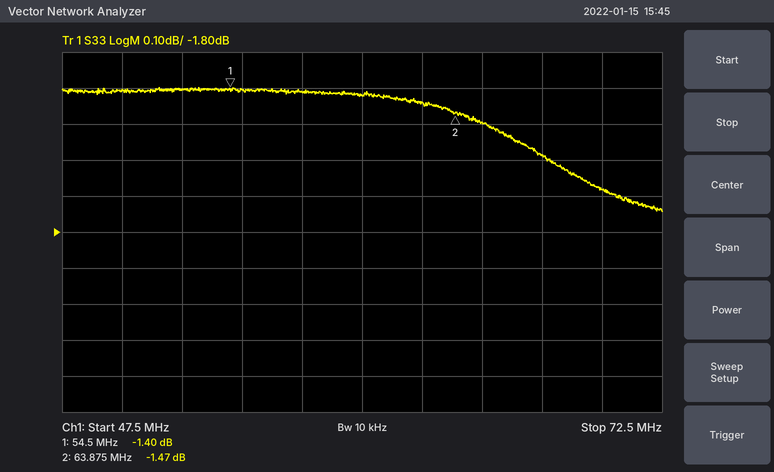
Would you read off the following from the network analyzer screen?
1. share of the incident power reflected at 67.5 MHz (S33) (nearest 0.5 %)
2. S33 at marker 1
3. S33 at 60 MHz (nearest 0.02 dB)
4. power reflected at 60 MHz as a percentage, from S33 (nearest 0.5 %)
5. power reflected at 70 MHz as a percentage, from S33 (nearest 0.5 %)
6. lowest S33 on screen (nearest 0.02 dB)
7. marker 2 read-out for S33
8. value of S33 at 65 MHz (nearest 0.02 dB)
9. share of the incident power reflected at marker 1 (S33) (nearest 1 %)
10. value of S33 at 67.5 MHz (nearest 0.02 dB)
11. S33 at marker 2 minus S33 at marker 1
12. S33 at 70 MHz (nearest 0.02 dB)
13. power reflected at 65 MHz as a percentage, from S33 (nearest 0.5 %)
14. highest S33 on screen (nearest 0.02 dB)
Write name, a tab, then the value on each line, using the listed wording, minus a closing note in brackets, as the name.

share of the incident power reflected at 67.5 MHz (S33)	69.5 %
S33 at marker 1	-1.40 dB
S33 at 60 MHz	-1.42 dB
power reflected at 60 MHz as a percentage, from S33	72.0 %
power reflected at 70 MHz as a percentage, from S33	68.0 %
lowest S33 on screen	-1.74 dB
marker 2 read-out for S33	-1.47 dB
value of S33 at 65 MHz	-1.50 dB
share of the incident power reflected at marker 1 (S33)	72 %
value of S33 at 67.5 MHz	-1.58 dB
S33 at marker 2 minus S33 at marker 1	-0.07 dB
S33 at 70 MHz	-1.68 dB
power reflected at 65 MHz as a percentage, from S33	71.0 %
highest S33 on screen	-1.40 dB
